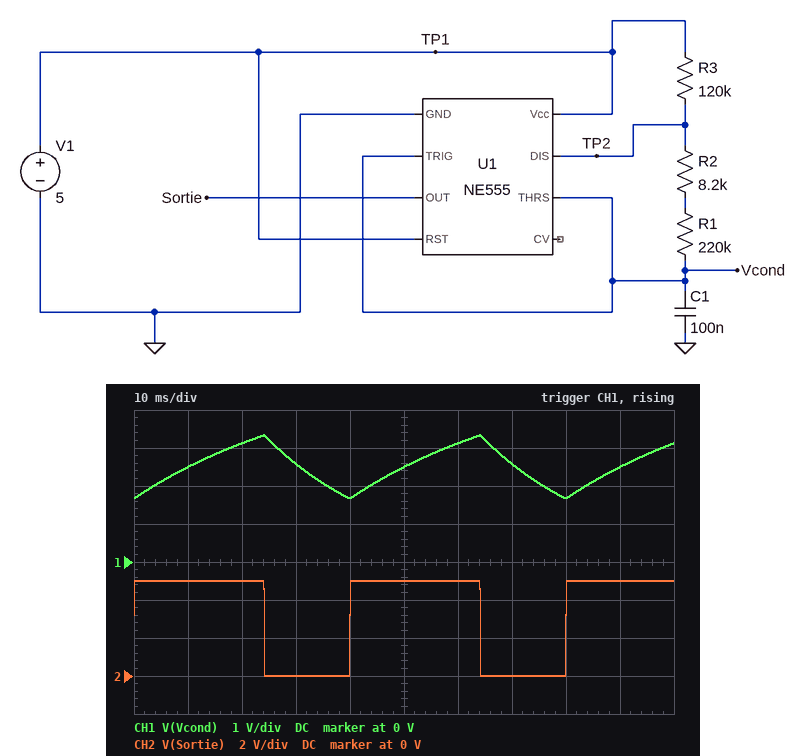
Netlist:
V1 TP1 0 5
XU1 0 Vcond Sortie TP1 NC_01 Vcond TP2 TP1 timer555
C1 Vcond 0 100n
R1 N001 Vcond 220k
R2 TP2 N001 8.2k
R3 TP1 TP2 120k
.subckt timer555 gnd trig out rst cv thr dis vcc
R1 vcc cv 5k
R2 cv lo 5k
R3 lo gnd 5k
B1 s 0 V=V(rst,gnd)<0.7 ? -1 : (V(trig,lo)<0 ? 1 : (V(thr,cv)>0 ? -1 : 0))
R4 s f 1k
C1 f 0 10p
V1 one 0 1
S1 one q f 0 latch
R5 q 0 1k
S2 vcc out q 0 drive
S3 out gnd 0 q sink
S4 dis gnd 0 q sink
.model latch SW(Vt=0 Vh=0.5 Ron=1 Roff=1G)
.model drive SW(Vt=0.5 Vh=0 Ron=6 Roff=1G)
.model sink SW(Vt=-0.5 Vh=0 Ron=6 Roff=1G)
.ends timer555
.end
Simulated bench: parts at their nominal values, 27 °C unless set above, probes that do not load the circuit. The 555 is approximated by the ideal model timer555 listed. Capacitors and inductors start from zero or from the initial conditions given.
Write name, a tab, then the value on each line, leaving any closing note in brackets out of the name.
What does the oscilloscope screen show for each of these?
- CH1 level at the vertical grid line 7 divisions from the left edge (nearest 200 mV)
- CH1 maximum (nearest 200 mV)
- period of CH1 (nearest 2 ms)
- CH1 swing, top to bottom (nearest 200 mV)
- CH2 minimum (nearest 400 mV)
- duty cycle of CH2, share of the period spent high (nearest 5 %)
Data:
CH1 level at the vertical grid line 7 divisions from the left edge	2.6 V
CH1 maximum	3.4 V
period of CH1	40 ms
CH1 swing, top to bottom	1.6 V
CH2 minimum	0 V
duty cycle of CH2, share of the period spent high	60 %
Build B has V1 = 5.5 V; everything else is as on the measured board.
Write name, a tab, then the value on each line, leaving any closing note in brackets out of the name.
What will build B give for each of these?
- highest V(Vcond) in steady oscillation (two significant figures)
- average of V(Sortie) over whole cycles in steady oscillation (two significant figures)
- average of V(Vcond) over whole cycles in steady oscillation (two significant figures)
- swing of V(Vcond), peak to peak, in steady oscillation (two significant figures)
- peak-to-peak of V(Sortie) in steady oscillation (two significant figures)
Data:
highest V(Vcond) in steady oscillation	3.7 V
average of V(Sortie) over whole cycles in steady oscillation	3.3 V
average of V(Vcond) over whole cycles in steady oscillation	2.8 V
swing of V(Vcond), peak to peak, in steady oscillation	1.8 V
peak-to-peak of V(Sortie) in steady oscillation	5.5 V
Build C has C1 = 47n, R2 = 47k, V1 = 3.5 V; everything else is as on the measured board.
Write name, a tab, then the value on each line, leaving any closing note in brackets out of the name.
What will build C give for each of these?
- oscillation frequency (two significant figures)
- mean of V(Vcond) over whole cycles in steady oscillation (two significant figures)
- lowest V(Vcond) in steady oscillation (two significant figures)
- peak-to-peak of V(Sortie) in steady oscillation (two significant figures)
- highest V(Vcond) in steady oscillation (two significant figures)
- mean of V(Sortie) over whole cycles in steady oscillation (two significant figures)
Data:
oscillation frequency	47 Hz
mean of V(Vcond) over whole cycles in steady oscillation	1.8 V
lowest V(Vcond) in steady oscillation	1.2 V
peak-to-peak of V(Sortie) in steady oscillation	3.5 V
highest V(Vcond) in steady oscillation	2.3 V
mean of V(Sortie) over whole cycles in steady oscillation	2.1 V
